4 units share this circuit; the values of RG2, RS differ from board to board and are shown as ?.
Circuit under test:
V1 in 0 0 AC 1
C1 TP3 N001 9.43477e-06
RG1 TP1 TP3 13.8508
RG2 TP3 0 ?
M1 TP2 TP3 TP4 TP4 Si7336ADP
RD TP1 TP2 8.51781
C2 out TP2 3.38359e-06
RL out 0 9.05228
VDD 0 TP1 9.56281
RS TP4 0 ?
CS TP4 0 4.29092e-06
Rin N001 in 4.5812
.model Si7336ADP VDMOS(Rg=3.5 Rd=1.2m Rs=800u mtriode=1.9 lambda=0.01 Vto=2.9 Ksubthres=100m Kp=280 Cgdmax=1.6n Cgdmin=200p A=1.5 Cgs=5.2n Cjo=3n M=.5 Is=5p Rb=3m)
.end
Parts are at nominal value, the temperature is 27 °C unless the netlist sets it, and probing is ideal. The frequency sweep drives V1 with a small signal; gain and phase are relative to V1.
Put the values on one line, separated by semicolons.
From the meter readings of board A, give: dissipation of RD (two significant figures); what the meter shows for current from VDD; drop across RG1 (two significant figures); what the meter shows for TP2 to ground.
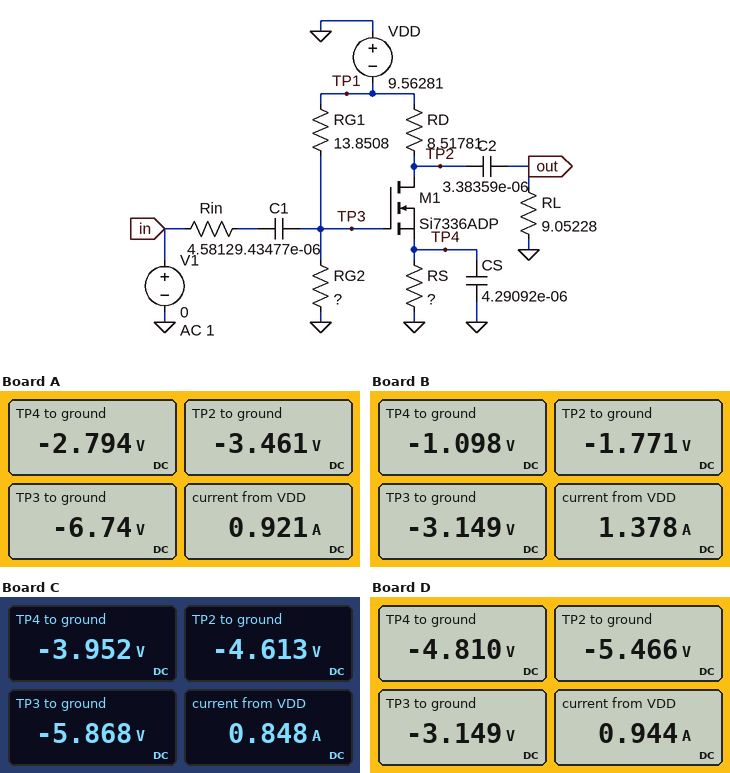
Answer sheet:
4.4 W; 0.921 A; 2.8 V; -3.461 V
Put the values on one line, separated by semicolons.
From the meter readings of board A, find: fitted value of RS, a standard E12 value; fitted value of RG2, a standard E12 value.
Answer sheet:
3.9 Ω; 33 Ω
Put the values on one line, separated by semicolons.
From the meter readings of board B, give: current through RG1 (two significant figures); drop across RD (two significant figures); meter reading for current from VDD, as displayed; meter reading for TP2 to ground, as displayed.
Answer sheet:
460 mA; 7.8 V; 1.378 A; -1.771 V
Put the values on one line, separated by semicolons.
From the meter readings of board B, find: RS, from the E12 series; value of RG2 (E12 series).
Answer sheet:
1.2 Ω; 6.8 Ω
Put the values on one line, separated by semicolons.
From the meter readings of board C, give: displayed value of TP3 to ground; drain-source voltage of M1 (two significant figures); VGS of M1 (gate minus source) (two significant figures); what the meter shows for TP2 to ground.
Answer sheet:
-5.868 V; -660 mV; -1.9 V; -4.613 V
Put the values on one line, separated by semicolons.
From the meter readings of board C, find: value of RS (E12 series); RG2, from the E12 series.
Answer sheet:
6.8 Ω; 22 Ω
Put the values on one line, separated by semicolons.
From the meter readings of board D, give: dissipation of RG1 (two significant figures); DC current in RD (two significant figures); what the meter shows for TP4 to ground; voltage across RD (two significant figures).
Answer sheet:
3.0 W; 480 mA; -4.810 V; 4.1 V
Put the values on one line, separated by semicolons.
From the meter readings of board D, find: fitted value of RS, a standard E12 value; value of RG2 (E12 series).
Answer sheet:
10 Ω; 6.8 Ω
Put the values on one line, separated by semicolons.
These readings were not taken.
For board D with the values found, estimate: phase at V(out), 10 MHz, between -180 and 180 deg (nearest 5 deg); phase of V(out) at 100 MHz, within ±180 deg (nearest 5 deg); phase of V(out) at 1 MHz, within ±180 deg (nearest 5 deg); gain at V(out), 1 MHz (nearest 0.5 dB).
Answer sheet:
5 deg; -10 deg; 5 deg; -62.0 dB
